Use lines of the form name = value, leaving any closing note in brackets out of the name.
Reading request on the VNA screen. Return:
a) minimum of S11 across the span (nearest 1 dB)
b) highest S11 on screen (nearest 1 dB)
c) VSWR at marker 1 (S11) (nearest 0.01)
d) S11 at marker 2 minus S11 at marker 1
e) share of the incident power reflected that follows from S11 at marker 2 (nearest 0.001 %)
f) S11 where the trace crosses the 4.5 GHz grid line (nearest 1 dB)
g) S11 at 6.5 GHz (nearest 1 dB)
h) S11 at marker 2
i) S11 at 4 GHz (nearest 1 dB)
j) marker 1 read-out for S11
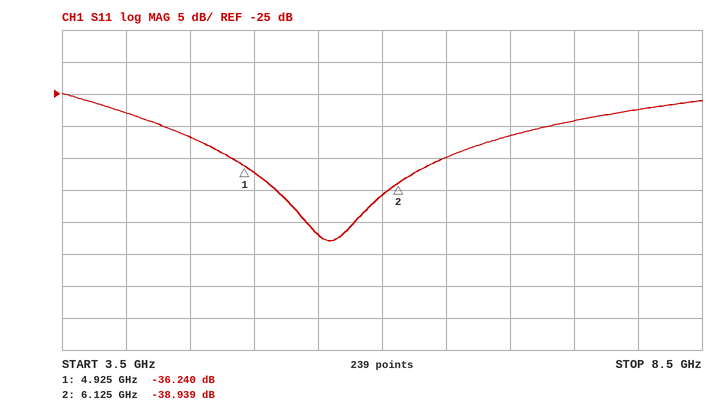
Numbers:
minimum of S11 across the span = -48 dB
highest S11 on screen = -25 dB
VSWR at marker 1 (S11) = 1.03
S11 at marker 2 minus S11 at marker 1 = -2.699 dB
share of the incident power reflected that follows from S11 at marker 2 = 0.013 %
S11 where the trace crosses the 4.5 GHz grid line = -32 dB
S11 at 6.5 GHz = -35 dB
S11 at marker 2 = -38.939 dB
S11 at 4 GHz = -28 dB
marker 1 read-out for S11 = -36.240 dB
